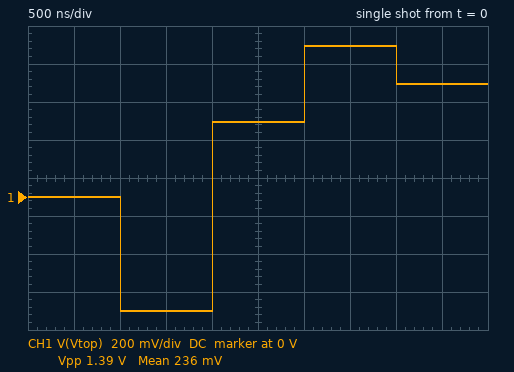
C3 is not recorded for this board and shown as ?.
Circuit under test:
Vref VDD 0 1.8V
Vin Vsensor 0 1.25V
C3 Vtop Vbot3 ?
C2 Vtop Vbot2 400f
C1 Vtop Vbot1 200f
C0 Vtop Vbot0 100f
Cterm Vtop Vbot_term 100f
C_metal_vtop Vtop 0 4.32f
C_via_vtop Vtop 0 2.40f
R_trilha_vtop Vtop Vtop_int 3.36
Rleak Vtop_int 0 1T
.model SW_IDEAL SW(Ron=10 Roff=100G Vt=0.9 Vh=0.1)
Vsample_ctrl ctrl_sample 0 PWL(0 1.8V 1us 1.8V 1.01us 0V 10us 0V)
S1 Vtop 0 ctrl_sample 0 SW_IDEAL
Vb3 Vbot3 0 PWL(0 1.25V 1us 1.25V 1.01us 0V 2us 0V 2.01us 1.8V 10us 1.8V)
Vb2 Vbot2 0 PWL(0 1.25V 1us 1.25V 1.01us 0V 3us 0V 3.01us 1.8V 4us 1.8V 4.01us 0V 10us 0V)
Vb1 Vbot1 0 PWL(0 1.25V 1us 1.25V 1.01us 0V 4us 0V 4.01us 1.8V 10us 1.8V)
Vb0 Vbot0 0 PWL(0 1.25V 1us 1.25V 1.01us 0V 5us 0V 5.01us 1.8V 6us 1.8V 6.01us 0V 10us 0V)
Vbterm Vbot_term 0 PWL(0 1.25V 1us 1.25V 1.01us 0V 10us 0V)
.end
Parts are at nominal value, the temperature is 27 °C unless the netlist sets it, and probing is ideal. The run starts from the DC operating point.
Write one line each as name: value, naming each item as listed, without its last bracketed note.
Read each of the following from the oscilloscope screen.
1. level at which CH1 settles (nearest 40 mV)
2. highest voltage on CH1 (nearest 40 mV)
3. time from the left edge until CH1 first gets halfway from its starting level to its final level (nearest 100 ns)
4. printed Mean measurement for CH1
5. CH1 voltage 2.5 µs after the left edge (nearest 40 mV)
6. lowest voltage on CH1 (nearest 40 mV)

level at which CH1 settles: 600 mV
highest voltage on CH1: 800 mV
time from the left edge until CH1 first gets halfway from its starting level to its final level: 2.0 µs
printed Mean measurement for CH1: 236 mV
CH1 voltage 2.5 µs after the left edge: 400 mV
lowest voltage on CH1: -600 mV
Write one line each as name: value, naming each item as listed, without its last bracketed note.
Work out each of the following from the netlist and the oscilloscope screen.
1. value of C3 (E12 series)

value of C3: 1 pF
